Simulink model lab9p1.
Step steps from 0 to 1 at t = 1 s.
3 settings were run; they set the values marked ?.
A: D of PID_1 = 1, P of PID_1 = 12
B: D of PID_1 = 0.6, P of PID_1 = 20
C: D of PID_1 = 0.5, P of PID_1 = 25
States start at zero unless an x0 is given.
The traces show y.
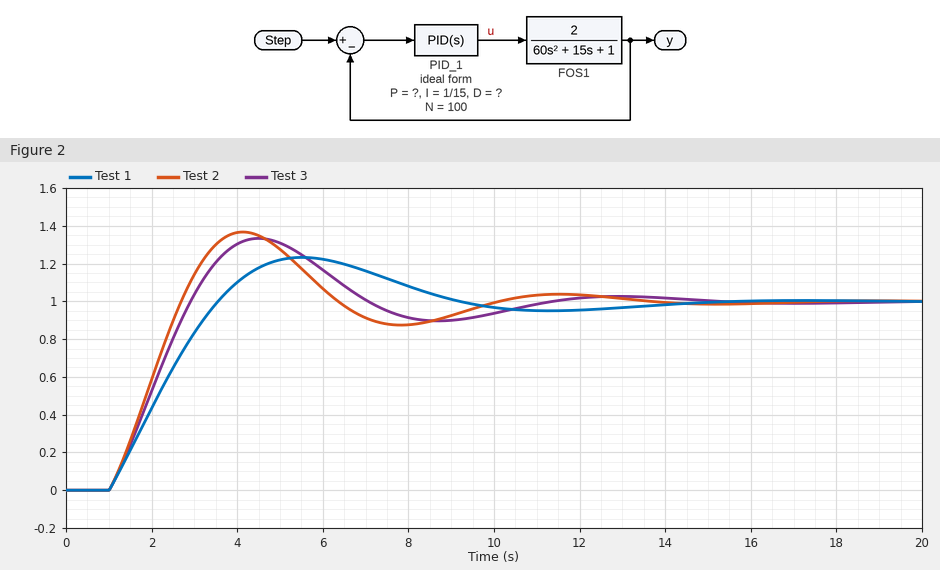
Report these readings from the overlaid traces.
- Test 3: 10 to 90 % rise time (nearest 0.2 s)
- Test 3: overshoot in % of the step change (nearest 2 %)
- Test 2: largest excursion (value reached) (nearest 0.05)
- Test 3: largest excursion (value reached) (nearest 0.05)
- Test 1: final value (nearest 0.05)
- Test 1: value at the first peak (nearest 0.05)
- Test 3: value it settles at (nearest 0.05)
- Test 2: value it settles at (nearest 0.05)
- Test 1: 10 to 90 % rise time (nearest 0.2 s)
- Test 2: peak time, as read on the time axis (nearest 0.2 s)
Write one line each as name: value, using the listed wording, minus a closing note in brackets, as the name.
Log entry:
Test 3: 10 to 90 % rise time: 1.4 s
Test 3: overshoot in % of the step change: 34 %
Test 2: largest excursion (value reached): 1.35
Test 3: largest excursion (value reached): 1.35
Test 1: final value: 1.00
Test 1: value at the first peak: 1.25
Test 3: value it settles at: 1.00
Test 2: value it settles at: 1.00
Test 1: 10 to 90 % rise time: 2.0 s
Test 2: peak time, as read on the time axis: 4.2 s
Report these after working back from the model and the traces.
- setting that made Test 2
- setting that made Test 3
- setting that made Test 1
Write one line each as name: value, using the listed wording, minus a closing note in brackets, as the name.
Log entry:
setting that made Test 2: C
setting that made Test 3: B
setting that made Test 1: A
